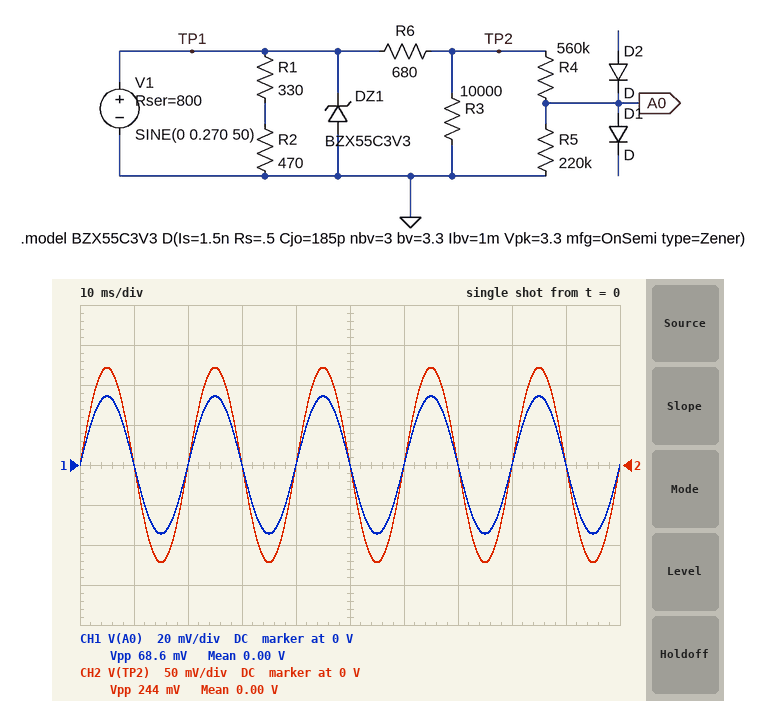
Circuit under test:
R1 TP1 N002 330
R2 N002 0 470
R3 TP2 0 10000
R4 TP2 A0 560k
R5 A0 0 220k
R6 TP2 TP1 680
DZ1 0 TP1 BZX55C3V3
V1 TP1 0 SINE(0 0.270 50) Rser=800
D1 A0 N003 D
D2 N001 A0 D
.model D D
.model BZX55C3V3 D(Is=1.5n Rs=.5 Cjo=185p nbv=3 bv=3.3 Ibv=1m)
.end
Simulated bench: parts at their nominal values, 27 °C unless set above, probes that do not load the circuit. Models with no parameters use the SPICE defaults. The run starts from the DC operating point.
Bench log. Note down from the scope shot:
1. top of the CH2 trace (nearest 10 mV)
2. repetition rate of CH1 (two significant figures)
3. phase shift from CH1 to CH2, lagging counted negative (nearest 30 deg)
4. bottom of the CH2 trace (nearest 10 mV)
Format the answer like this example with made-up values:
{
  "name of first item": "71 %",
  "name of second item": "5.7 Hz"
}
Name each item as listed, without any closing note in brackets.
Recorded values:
{
  "top of the CH2 trace": "120 mV",
  "repetition rate of CH1": "50 Hz",
  "phase shift from CH1 to CH2, lagging counted negative": "0 deg",
  "bottom of the CH2 trace": "-120 mV"
}
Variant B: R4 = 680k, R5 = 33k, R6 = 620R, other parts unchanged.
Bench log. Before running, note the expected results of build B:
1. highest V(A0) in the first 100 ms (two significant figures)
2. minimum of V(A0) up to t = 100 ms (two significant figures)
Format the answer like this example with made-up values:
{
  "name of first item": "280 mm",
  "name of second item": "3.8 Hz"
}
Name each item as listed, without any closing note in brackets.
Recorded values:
{
  "highest V(A0) in the first 100 ms": "5.7 mV",
  "minimum of V(A0) up to t = 100 ms": "-5.7 mV"
}
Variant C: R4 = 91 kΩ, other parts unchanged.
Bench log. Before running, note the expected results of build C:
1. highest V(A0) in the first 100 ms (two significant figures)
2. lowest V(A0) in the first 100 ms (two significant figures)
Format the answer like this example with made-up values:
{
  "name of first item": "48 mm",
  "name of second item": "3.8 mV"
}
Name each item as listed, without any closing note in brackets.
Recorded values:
{
  "highest V(A0) in the first 100 ms": "86 mV",
  "lowest V(A0) in the first 100 ms": "-86 mV"
}
